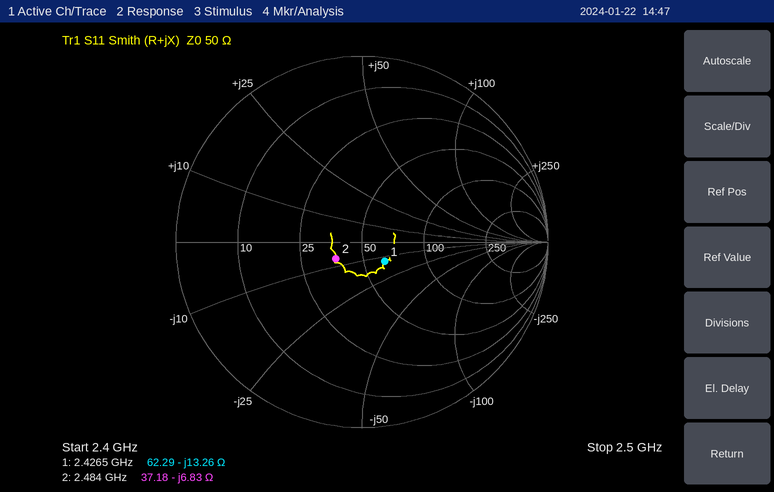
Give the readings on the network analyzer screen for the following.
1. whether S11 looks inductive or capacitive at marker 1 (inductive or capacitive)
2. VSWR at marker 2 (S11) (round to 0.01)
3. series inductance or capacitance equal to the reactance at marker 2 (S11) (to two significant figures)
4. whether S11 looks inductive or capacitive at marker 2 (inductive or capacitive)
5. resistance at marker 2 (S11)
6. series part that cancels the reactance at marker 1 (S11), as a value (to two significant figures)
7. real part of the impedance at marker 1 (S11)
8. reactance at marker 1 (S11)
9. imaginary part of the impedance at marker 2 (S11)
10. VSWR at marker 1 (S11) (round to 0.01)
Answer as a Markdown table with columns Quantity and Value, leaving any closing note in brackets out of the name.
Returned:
| Quantity | Value |
|---|---|
| whether S11 looks inductive or capacitive at marker 1 | capacitive |
| VSWR at marker 2 (S11) | 1.40 |
| series inductance or capacitance equal to the reactance at marker 2 (S11) | 9.4 pF |
| whether S11 looks inductive or capacitive at marker 2 | capacitive |
| resistance at marker 2 | 37.18 Ω |
| series part that cancels the reactance at marker 1 (S11), as a value | 870 pH |
| real part of the impedance at marker 1 | 62.29 Ω |
| reactance at marker 1 | -13.26 Ω |
| imaginary part of the impedance at marker 2 | -6.83 Ω |
| VSWR at marker 1 (S11) | 1.38 |
